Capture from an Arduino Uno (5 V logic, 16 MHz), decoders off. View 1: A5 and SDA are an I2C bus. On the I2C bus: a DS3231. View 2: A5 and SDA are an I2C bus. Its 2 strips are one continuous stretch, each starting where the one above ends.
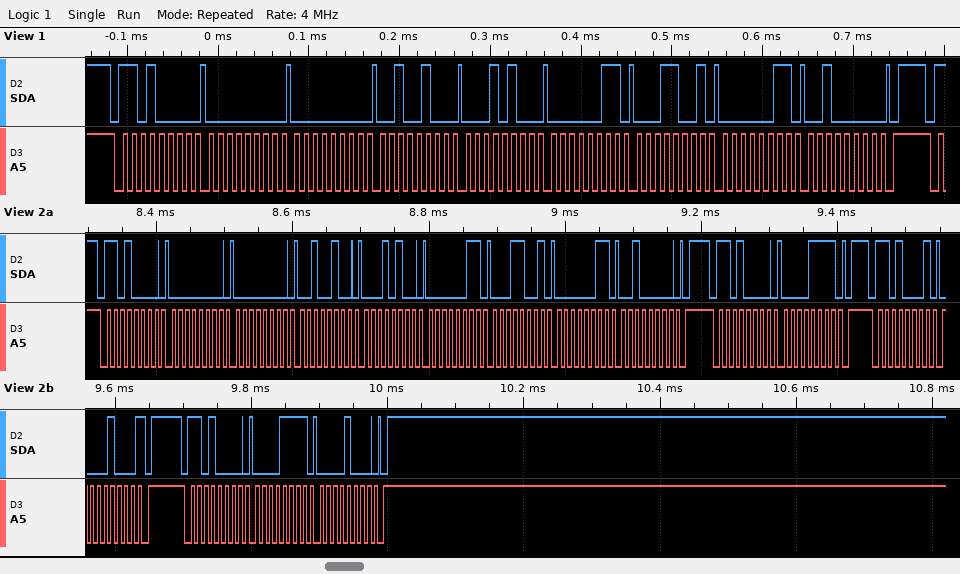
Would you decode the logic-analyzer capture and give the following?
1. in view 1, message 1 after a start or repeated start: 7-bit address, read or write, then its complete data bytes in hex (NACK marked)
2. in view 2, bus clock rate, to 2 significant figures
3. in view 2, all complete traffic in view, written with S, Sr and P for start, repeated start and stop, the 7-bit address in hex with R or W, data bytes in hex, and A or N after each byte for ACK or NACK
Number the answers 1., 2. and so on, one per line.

1. 0x68 write: 00 00 24 14 03 19 03 20
2. 100 kHz
3. S 68W A 00 A 00 A 24 A 14 A 03 A 19 A 03 A 20 A P S 68W A 0F A P S 68R A 08 N P S 68W A 0F A 08 A P
